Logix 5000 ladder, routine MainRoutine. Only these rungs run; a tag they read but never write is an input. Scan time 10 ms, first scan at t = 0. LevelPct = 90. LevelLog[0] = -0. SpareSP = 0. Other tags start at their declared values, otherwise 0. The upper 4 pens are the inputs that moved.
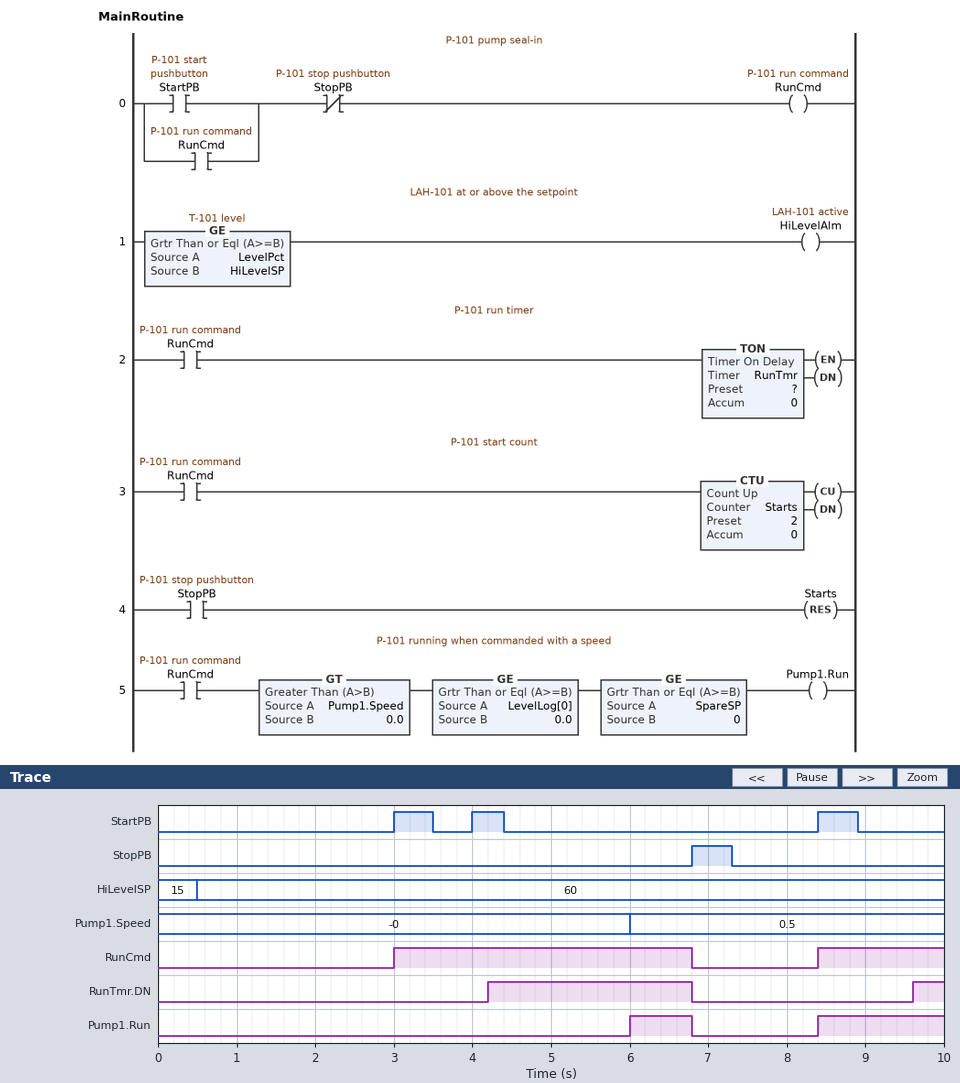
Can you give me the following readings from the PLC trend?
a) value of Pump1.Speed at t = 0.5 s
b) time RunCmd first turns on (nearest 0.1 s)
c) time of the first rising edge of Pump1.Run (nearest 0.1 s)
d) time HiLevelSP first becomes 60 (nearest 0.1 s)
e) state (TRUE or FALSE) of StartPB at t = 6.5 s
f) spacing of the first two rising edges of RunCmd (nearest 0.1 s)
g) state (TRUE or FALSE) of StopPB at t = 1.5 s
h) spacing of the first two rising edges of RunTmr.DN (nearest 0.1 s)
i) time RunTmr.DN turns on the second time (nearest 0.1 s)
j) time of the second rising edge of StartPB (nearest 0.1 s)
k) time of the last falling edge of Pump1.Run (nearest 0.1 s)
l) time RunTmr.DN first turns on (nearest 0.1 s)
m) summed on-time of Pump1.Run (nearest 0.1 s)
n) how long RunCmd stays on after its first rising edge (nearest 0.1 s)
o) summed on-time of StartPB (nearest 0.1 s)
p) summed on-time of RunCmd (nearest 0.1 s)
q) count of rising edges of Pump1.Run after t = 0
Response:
-0
3.0 s
6.0 s
0.5 s
FALSE
5.4 s
FALSE
5.4 s
9.6 s
4.0 s
6.8 s
4.2 s
2.4 s
3.8 s
1.4 s
5.4 s
2
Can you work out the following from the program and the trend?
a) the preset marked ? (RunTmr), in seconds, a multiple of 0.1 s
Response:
1.2 s
